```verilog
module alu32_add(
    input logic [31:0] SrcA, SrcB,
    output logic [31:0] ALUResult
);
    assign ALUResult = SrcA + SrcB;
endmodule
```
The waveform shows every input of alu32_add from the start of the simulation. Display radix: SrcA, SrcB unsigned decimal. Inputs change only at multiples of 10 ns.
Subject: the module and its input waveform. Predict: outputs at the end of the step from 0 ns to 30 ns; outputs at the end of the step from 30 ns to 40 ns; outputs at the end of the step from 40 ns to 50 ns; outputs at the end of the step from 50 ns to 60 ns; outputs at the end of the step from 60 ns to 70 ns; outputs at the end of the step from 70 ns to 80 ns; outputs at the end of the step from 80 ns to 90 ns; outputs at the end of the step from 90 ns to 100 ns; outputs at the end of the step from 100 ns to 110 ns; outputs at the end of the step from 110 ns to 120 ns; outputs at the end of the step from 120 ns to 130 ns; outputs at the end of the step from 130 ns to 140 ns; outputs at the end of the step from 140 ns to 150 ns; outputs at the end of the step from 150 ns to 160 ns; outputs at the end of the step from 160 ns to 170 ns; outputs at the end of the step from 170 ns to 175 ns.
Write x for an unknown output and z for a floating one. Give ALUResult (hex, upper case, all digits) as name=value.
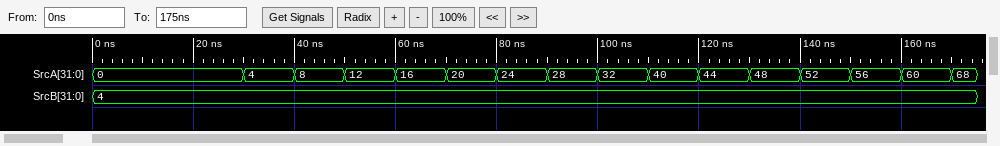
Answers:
ALUResult=00000004
ALUResult=00000008
ALUResult=0000000C
ALUResult=00000010
ALUResult=00000014
ALUResult=00000018
ALUResult=0000001C
ALUResult=00000020
ALUResult=00000024
ALUResult=0000002C
ALUResult=00000030
ALUResult=00000034
ALUResult=00000038
ALUResult=0000003C
ALUResult=00000040
ALUResult=00000048
